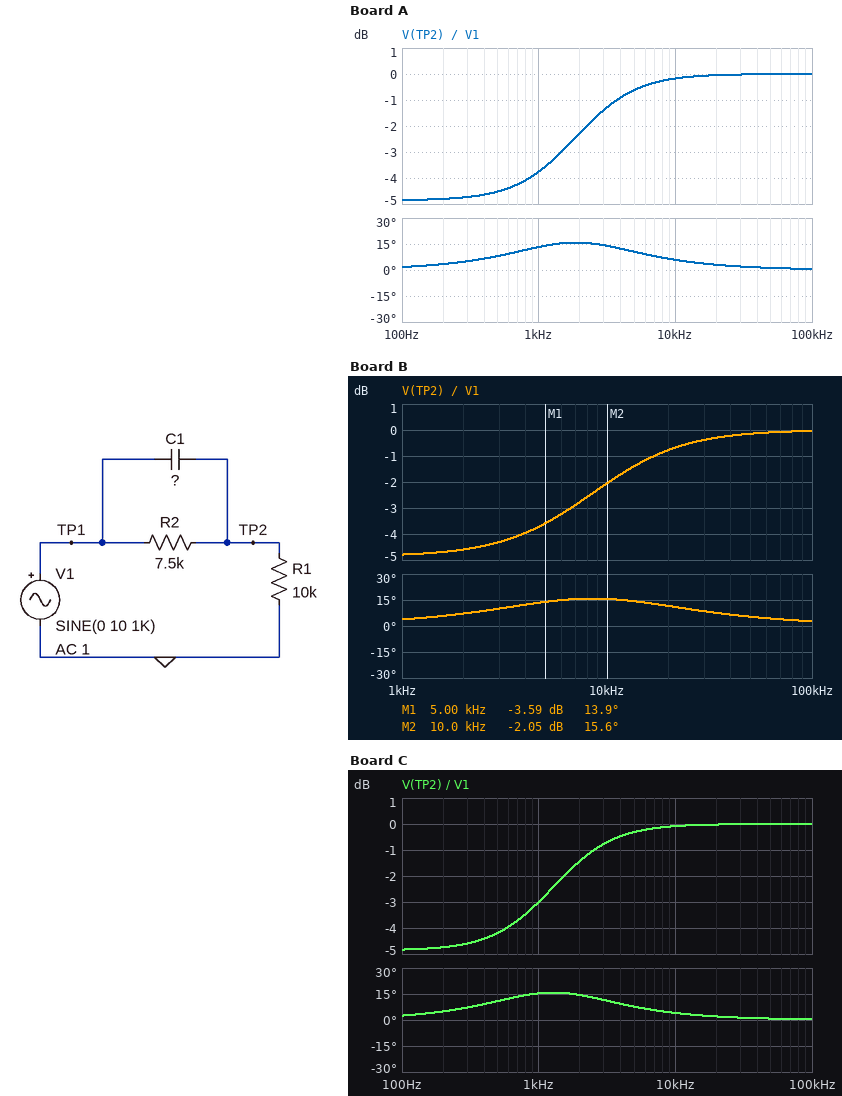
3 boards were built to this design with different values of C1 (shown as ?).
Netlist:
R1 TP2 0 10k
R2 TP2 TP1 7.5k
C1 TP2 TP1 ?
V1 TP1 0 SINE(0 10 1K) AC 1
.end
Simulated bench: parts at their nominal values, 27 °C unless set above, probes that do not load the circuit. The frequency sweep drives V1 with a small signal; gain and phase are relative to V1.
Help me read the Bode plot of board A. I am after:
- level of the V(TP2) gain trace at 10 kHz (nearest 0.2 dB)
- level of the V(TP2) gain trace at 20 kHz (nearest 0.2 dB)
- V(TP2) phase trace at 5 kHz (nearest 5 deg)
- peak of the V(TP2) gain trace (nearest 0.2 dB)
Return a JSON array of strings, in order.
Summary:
["-0.2 dB", "0 dB", "10 deg", "0 dB"]
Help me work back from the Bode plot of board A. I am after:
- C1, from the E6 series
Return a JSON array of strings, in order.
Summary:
["15 nF"]
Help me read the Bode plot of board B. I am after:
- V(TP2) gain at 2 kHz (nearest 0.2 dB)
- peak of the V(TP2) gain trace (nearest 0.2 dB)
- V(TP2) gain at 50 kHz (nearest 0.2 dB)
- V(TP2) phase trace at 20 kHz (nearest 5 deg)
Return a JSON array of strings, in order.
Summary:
["-4.6 dB", "0 dB", "-0.2 dB", "10 deg"]
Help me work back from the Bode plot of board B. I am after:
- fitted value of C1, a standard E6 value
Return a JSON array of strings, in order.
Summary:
["3.3 nF"]
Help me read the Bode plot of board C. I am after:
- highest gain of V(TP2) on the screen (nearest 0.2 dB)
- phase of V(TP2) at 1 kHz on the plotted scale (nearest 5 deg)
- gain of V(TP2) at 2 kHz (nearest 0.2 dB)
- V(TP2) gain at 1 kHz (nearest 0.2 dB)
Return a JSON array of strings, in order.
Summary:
["0 dB", "15 deg", "-1.4 dB", "-3.0 dB"]
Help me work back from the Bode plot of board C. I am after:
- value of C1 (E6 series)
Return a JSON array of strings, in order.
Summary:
["22 nF"]
